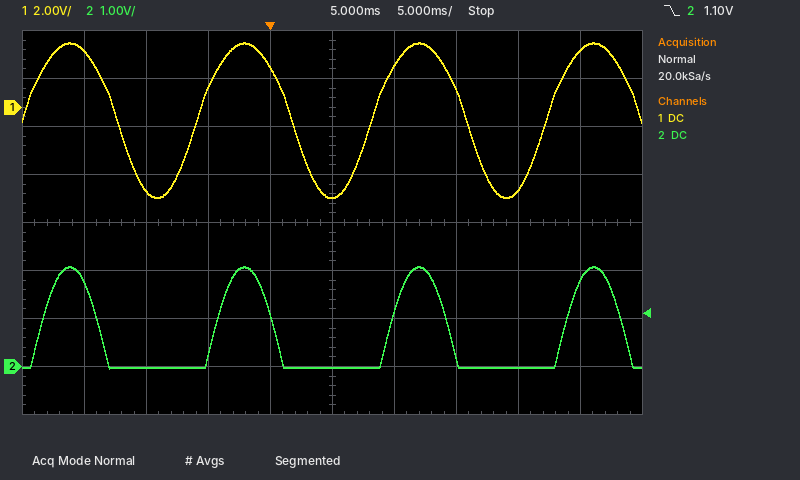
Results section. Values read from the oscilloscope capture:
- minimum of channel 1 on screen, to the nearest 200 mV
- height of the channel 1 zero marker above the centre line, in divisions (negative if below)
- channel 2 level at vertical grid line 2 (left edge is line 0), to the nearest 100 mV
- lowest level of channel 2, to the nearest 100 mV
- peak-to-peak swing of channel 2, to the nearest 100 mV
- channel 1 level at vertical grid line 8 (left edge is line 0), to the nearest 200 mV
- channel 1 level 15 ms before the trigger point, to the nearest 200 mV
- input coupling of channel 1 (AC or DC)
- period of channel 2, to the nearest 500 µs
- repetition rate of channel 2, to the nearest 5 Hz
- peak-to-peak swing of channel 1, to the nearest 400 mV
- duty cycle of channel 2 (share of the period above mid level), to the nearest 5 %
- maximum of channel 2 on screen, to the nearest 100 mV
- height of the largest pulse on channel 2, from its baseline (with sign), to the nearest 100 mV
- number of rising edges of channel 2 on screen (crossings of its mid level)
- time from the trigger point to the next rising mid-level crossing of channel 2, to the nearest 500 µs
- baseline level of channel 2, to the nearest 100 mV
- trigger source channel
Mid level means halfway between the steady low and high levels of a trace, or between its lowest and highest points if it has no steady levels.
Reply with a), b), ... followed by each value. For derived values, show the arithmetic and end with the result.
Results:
a) -3.8 V
b) +2.4 div
c) 0.0 V
d) 0.0 V
e) 2.1 V − (0.0 V) = 2.1 V
f) -3.4 V
g) 2.4 V
h) DC
i) 14.0 ms
j) 1 / 14.0 ms ≈ 71.4 Hz, so 70 Hz to the nearest 5 Hz
k) 6.4 V
l) 30 %
m) 2.1 V
n) 2.1 V − (0.0 V) = +2.1 V
o) 4
p) 10.0 ms
q) 0.0 V
r) channel 2
